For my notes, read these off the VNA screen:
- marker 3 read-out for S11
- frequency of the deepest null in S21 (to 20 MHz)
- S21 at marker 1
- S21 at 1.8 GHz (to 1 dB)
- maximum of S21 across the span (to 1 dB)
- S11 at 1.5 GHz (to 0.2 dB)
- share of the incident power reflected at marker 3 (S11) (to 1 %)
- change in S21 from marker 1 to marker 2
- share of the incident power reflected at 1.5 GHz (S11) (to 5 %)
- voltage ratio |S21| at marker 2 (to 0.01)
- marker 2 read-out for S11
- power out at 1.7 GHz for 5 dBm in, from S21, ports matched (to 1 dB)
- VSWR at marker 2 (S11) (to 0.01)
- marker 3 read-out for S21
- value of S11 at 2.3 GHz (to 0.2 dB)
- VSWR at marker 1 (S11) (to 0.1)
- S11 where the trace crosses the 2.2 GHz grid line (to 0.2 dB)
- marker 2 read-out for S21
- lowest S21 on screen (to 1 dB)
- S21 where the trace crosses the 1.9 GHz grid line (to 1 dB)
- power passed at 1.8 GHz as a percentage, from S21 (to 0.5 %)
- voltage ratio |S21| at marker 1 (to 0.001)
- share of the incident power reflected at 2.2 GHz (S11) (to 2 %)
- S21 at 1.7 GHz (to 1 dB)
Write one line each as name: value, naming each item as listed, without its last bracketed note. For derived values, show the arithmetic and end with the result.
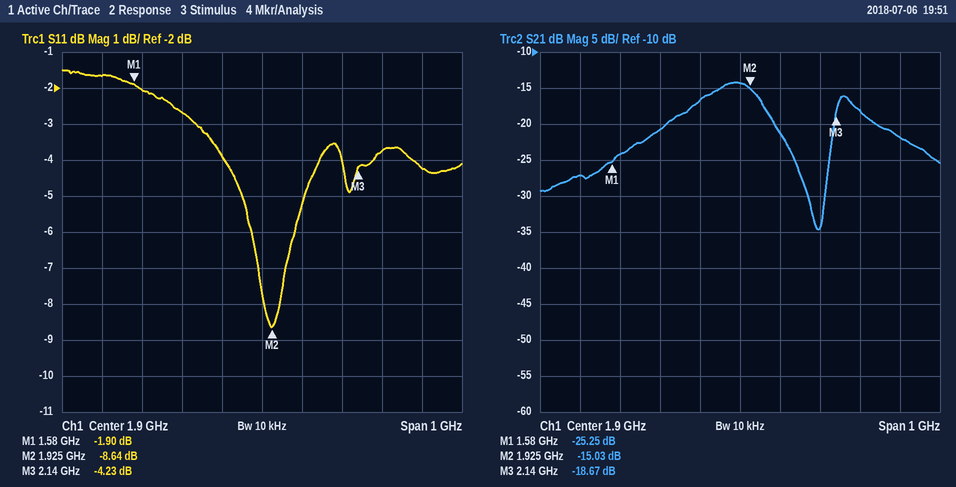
marker 3 read-out for S11: -4.23 dB
frequency of the deepest null in S21: 2.10 GHz
S21 at marker 1: -25.25 dB
S21 at 1.8 GHz: -17 dB
maximum of S21 across the span: -14 dB
S11 at 1.5 GHz: -1.6 dB
share of the incident power reflected at marker 3 (S11): 10^(-4.23/10) ≈ 38 %
change in S21 from marker 1 to marker 2: -15.03 − (-25.25) = 10.22 dB
share of the incident power reflected at 1.5 GHz (S11): 10^(-1.6/10) ≈ 69.2 %, so 70 % to the nearest 5 %
voltage ratio |S21| at marker 2: 10^(-15.03/20) ≈ 0.18
marker 2 read-out for S11: -8.64 dB
power out at 1.7 GHz for 5 dBm in, from S21, ports matched: 5 dBm + (-21 dB) = -16 dBm
VSWR at marker 2 (S11): (1 + 0.3698)/(1 − 0.3698) ≈ 2.17
marker 3 read-out for S21: -18.67 dB
value of S11 at 2.3 GHz: -4.2 dB
VSWR at marker 1 (S11): (1 + 0.8035)/(1 − 0.8035) ≈ 9.2
S11 where the trace crosses the 2.2 GHz grid line: -3.8 dB
marker 2 read-out for S21: -15.03 dB
lowest S21 on screen: -35 dB
S21 where the trace crosses the 1.9 GHz grid line: -14 dB
power passed at 1.8 GHz as a percentage, from S21: 10^(-17/10) ≈ 2.0 %
voltage ratio |S21| at marker 1: 10^(-25.25/20) ≈ 0.055
share of the incident power reflected at 2.2 GHz (S11): 10^(-3.8/10) ≈ 42 %
S21 at 1.7 GHz: -21 dB
